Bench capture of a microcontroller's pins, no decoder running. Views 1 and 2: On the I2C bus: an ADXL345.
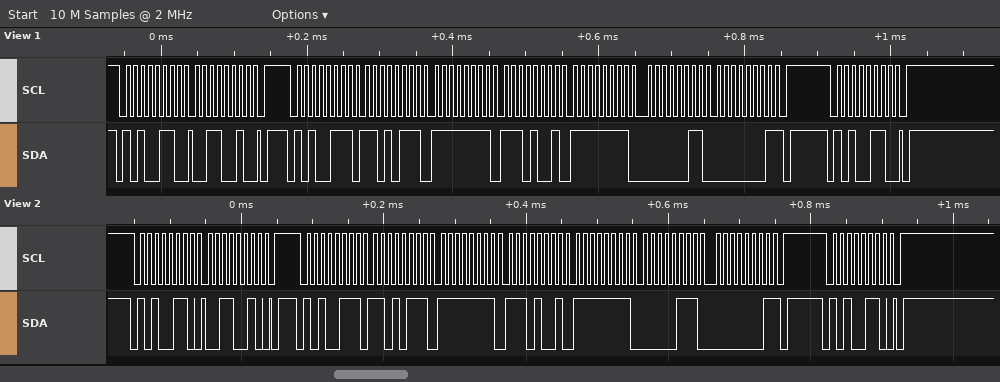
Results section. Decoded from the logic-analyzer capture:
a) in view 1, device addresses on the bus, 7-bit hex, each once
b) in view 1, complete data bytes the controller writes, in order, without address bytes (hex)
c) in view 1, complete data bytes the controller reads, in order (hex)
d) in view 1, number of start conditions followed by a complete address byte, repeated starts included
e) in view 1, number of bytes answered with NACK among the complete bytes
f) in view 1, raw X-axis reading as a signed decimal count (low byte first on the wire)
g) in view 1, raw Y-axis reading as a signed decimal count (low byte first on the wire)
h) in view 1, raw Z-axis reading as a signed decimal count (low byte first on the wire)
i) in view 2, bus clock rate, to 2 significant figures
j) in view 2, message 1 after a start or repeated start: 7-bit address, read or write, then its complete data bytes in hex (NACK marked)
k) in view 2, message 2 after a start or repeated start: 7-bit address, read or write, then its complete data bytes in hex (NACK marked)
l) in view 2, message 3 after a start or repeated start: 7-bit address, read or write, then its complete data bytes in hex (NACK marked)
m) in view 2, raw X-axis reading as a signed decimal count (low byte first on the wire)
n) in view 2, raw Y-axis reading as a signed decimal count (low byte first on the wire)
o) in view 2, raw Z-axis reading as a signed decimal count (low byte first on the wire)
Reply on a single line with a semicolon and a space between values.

0x53; 32; D7 FF E9 FF 03 01; 3; 1; -41; -23; 259; 100 kHz; 0x53 write: 32; 0x53 read: D7 FF E9 FF 07 01 NACK; 0x53 write; -41; -23; 263
